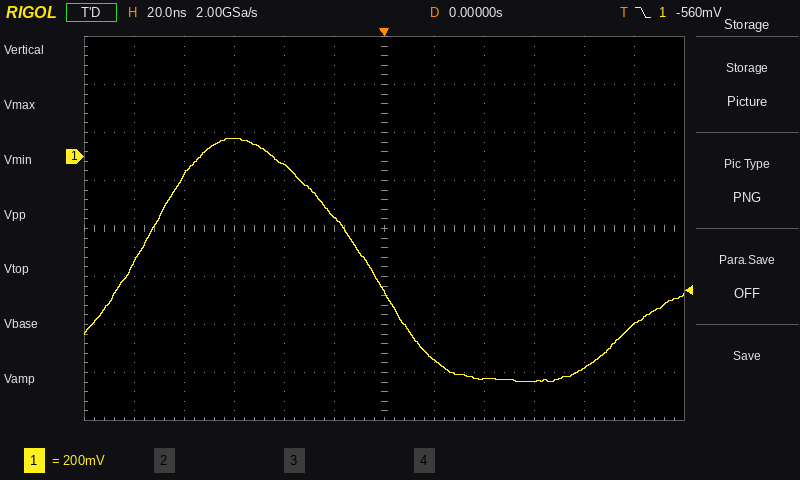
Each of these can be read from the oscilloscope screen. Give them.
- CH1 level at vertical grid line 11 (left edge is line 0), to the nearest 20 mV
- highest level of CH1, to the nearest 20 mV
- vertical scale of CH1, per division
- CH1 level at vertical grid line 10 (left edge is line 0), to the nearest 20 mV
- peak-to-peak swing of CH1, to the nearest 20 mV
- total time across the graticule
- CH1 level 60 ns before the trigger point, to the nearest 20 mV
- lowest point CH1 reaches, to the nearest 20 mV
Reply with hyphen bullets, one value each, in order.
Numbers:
- -700 mV
- 80 mV
- 200 mV
- -880 mV
- 1.02 V
- 240 ns
- 80 mV
- -940 mV
